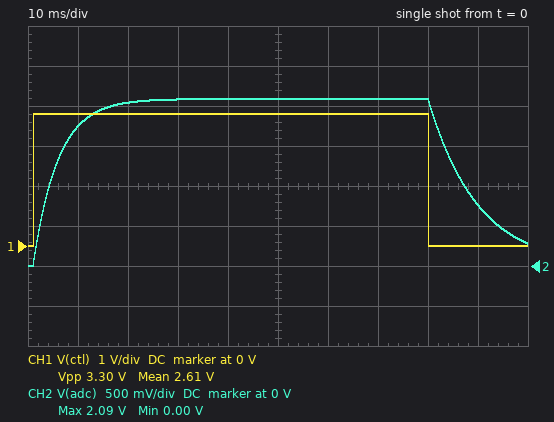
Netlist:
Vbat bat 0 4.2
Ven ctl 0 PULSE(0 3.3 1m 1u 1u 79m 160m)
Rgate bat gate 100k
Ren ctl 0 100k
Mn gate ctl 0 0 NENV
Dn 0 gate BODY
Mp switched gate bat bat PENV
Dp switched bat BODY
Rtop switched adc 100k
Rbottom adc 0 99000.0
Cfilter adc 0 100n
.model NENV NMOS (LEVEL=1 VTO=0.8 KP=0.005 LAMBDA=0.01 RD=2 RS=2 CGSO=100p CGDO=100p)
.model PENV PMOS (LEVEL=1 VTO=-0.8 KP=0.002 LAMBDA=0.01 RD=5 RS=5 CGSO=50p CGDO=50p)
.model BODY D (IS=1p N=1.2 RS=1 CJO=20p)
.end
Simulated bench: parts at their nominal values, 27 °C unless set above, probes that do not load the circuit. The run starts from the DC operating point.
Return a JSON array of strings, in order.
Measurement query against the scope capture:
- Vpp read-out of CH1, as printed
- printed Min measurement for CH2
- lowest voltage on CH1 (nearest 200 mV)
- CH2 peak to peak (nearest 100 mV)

["3.30 V", "0.00 V", "0 V", "2.1 V"]
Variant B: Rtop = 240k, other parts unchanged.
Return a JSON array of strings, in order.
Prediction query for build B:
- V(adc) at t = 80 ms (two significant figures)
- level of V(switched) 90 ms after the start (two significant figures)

["1.2 V", "450 mV"]
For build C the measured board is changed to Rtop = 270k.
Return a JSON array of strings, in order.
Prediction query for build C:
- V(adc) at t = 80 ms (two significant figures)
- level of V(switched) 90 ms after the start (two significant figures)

["1.1 V", "410 mV"]
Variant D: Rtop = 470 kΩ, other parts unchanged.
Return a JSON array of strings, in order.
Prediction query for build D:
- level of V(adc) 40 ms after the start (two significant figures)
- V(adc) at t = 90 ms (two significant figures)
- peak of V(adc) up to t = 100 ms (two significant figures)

["720 mV", "270 mV", "730 mV"]
